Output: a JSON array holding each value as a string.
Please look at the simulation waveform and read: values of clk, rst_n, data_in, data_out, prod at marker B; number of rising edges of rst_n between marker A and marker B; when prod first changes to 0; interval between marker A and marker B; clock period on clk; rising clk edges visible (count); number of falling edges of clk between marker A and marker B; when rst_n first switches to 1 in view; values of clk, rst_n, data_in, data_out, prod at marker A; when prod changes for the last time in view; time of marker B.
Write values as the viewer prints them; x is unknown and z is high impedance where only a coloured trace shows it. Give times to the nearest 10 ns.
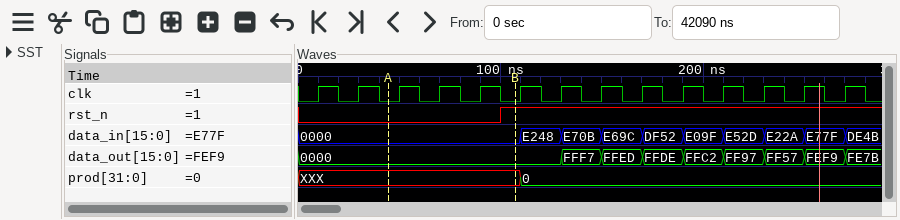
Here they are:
["clk=0, rst_n=1, data_in=0000, data_out=0000, prod=XXX", "1", "110 ns", "60 ns", "20 ns", "14", "3", "100 ns", "clk=0, rst_n=0, data_in=0000, data_out=0000, prod=XXX", "110 ns", "110 ns"]
